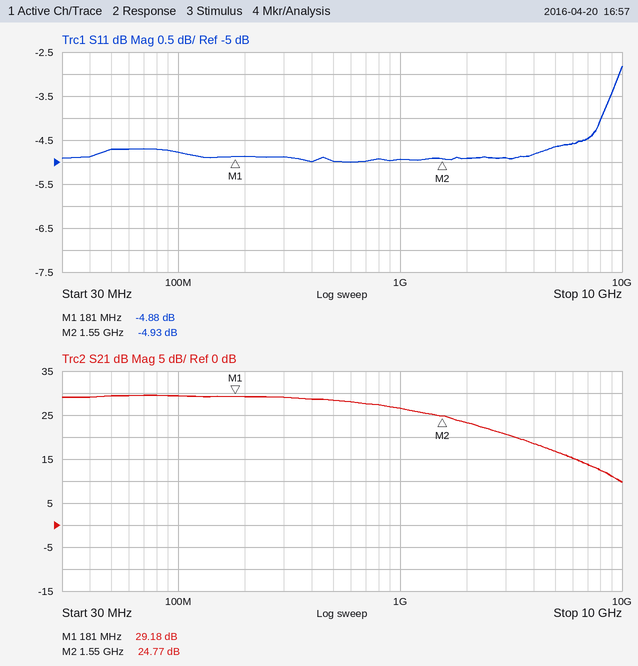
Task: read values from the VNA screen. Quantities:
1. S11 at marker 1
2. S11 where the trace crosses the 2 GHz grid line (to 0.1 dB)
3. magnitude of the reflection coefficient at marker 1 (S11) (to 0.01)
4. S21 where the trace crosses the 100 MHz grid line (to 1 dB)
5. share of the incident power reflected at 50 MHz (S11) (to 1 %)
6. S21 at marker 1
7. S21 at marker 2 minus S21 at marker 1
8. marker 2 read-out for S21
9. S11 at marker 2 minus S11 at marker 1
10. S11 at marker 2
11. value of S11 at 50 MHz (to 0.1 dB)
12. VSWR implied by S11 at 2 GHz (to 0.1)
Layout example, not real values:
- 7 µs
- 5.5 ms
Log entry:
- -4.88 dB
- -4.9 dB
- 0.57
- 29 dB
- 34 %
- 29.18 dB
- -4.41 dB
- 24.77 dB
- -0.05 dB
- -4.93 dB
- -4.7 dB
- 3.6
